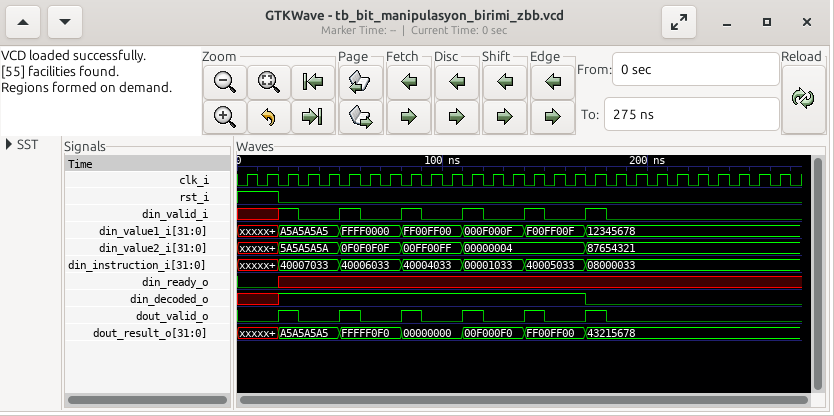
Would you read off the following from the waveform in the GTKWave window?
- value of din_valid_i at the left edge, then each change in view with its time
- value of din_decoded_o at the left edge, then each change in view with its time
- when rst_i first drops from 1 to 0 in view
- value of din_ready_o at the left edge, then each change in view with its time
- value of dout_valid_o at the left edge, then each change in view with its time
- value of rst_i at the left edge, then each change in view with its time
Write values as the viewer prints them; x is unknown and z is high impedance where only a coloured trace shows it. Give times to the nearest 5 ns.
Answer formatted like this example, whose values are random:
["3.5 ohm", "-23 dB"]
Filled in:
["x, 1 at 20 ns, 0 at 30 ns, 1 at 50 ns, 0 at 60 ns, 1 at 80 ns, 0 at 90 ns, 1 at 110 ns, 0 at 120 ns, 1 at 140 ns, 0 at 150 ns, 1 at 170 ns, 0 at 180 ns", "x, 1 at 20 ns, 0 at 170 ns", "20 ns", "0, x at 20 ns", "0, 1 at 20 ns, 0 at 30 ns, 1 at 50 ns, 0 at 60 ns, 1 at 80 ns, 0 at 90 ns, 1 at 110 ns, 0 at 120 ns, 1 at 140 ns, 0 at 150 ns, 1 at 170 ns, 0 at 180 ns", "1, 0 at 20 ns"]
